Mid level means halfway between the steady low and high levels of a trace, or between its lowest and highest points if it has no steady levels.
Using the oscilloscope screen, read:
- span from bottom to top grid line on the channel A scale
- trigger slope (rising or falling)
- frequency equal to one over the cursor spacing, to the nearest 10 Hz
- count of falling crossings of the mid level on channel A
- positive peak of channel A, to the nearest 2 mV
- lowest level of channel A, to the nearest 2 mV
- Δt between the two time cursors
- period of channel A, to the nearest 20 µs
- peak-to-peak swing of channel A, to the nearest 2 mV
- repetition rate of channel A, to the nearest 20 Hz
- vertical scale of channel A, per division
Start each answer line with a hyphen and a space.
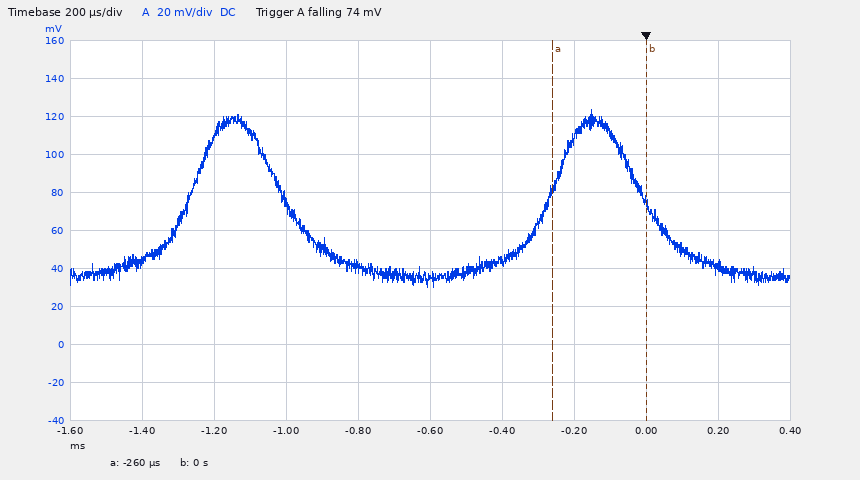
- 200 mV
- falling
- 3.85 kHz
- 2
- 124 mV
- 30 mV
- 260 µs
- 1.00 ms
- 94 mV
- 1.00 kHz
- 20 mV
